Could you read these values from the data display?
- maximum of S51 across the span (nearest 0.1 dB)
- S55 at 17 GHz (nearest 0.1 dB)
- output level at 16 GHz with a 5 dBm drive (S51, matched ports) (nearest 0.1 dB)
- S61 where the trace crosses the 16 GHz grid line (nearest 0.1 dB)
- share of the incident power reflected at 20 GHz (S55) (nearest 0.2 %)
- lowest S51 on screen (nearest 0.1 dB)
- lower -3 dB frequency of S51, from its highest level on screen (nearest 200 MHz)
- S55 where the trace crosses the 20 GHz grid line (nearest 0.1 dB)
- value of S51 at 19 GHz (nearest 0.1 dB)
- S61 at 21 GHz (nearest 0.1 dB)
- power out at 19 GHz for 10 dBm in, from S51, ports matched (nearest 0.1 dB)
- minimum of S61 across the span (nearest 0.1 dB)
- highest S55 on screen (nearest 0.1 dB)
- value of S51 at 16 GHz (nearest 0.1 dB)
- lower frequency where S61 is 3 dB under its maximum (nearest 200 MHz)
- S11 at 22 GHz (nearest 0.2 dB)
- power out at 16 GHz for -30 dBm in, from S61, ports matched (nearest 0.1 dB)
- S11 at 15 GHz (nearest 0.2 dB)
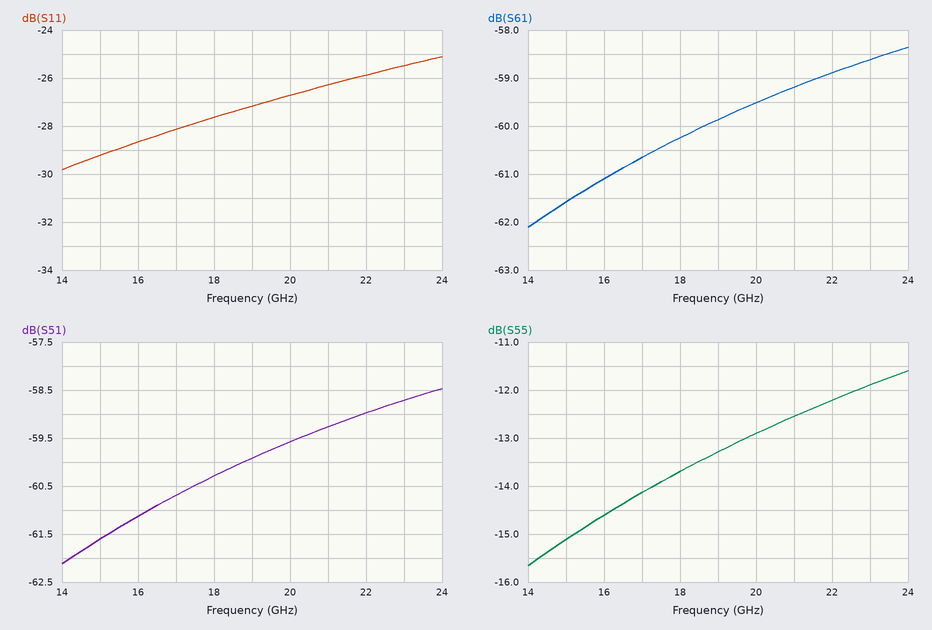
-58.5 dB
-14.1 dB
-56.1 dBm
-61.1 dB
5.2 %
-62.1 dB
15.2 GHz
-12.9 dB
-59.9 dB
-59.2 dB
-49.9 dBm
-62.1 dB
-11.6 dB
-61.1 dB
15.4 GHz
-25.8 dB
-91.1 dBm
-29.2 dB
